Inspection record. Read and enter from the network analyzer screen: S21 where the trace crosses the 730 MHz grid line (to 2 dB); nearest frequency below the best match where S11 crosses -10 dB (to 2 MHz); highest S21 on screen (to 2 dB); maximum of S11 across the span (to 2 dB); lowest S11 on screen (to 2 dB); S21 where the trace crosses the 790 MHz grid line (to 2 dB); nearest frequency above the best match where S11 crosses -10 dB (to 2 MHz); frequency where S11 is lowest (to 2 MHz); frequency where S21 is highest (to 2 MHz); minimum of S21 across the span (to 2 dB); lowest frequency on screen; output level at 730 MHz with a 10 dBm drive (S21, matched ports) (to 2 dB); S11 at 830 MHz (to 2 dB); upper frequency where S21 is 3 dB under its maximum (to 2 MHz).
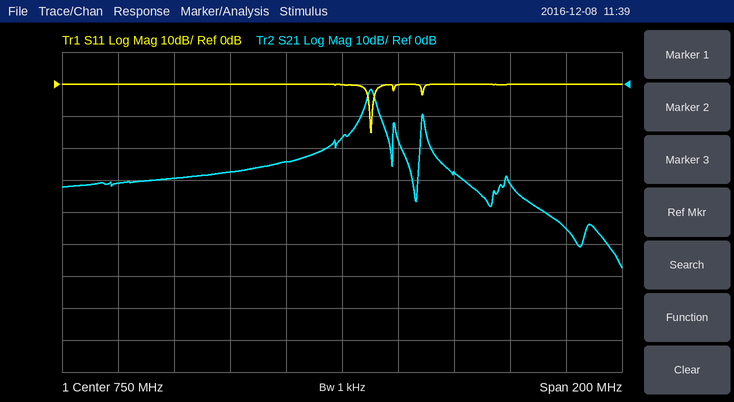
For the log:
-24 dB
760 MHz
-2 dB
0 dB
-16 dB
-28 dB
760 MHz
760 MHz
760 MHz
-58 dB
650 MHz
-14 dBm
0 dB
762 MHz
